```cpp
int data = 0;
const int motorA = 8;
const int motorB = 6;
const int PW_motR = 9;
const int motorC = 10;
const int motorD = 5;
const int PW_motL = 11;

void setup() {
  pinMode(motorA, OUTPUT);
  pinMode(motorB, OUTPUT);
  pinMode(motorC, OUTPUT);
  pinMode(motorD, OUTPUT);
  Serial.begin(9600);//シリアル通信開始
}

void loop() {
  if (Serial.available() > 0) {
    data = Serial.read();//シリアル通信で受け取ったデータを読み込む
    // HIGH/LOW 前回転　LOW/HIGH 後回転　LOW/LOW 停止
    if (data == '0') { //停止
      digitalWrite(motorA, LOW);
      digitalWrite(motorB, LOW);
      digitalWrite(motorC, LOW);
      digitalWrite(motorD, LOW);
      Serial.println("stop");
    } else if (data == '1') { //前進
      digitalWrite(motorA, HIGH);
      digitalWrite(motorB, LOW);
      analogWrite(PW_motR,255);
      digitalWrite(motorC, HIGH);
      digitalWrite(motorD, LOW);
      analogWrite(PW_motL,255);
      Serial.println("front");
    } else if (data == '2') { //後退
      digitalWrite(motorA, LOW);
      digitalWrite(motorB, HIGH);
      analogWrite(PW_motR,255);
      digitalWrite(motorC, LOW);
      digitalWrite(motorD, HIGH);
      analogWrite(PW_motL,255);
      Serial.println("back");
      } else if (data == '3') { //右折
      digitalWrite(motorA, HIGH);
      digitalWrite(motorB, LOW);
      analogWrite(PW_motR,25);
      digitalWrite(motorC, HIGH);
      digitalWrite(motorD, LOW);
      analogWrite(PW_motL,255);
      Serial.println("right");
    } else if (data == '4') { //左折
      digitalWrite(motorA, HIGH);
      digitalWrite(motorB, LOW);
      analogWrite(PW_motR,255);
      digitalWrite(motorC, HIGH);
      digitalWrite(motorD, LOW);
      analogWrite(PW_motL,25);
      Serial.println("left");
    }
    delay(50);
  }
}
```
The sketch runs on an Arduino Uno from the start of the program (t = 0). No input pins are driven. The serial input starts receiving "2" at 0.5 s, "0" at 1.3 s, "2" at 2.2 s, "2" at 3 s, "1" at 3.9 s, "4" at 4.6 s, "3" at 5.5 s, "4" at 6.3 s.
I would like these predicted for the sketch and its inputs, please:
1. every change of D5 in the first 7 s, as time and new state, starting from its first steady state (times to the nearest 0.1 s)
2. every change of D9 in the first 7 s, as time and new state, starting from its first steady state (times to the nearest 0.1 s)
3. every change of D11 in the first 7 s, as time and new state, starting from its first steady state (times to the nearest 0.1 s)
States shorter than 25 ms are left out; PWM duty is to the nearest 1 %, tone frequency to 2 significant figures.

0 s low; 0.5 s high; 1.3 s low; 2.2 s high; 3.9 s low
0.5 s high; 5.5 s PWM 10 %; 6.3 s high
0.5 s high; 4.6 s PWM 10 %; 5.5 s high; 6.3 s PWM 10 %
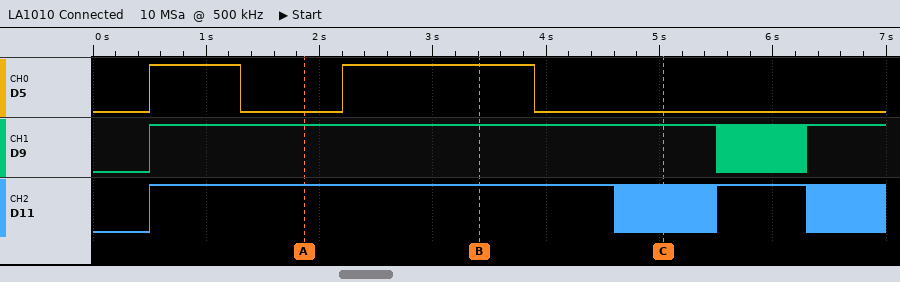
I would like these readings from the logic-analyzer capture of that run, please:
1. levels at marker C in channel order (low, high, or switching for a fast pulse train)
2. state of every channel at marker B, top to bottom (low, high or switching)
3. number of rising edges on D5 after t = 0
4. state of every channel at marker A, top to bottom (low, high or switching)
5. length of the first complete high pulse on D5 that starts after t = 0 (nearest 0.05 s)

D5 low, D9 high, D11 switching
D5 high, D9 high, D11 high
2
D5 low, D9 high, D11 high
0.80 s
